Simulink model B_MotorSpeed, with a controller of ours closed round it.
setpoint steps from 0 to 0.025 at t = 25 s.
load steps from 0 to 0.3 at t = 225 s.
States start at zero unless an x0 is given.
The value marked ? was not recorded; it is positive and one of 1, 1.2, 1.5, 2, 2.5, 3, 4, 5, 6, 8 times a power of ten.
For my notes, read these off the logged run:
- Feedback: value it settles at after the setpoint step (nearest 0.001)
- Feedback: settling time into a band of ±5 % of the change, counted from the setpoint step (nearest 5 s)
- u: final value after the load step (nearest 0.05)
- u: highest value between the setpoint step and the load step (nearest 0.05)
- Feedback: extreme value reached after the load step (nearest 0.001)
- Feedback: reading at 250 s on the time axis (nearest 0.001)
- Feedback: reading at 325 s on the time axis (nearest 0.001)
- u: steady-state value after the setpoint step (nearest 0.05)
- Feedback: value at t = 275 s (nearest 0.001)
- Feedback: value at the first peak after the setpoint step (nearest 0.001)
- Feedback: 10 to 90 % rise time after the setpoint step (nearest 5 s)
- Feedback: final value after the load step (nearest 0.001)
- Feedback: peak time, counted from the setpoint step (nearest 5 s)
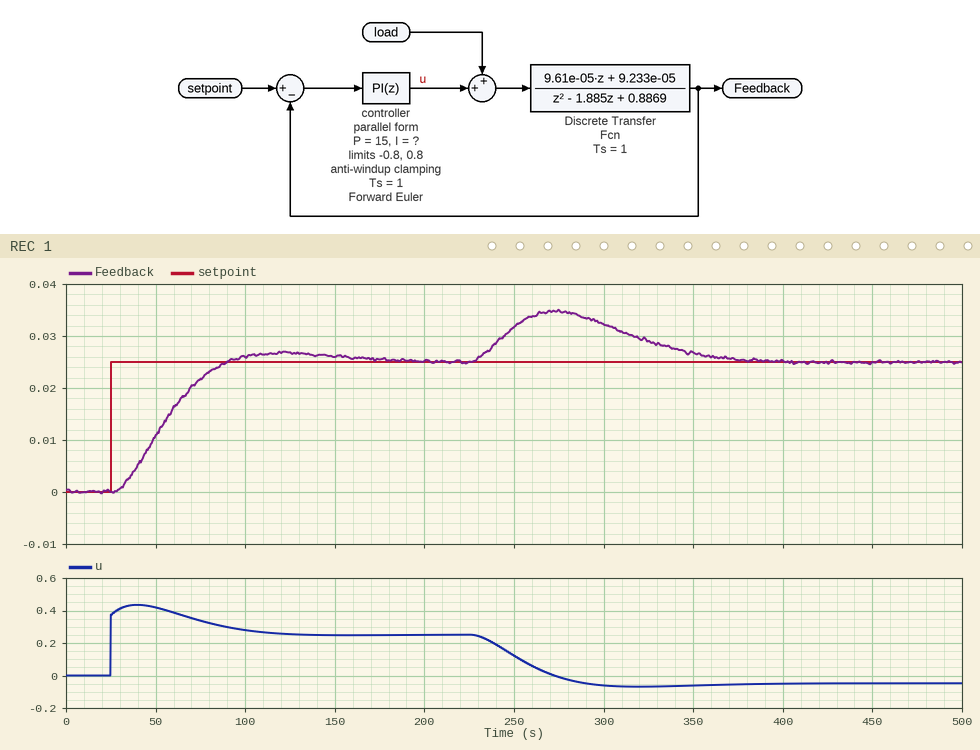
0.025
120 s
-0.05
0.45
0.035
0.032
0.029
0.25
0.035
0.027
45 s
0.025
95 s
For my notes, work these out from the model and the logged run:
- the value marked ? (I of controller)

0.4
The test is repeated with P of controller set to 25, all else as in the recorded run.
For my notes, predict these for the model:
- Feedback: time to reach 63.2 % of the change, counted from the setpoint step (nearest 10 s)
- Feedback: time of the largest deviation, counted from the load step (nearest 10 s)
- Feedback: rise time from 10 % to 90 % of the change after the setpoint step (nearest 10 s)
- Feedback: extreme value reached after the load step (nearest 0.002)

30 s
40 s
30 s
0.032
